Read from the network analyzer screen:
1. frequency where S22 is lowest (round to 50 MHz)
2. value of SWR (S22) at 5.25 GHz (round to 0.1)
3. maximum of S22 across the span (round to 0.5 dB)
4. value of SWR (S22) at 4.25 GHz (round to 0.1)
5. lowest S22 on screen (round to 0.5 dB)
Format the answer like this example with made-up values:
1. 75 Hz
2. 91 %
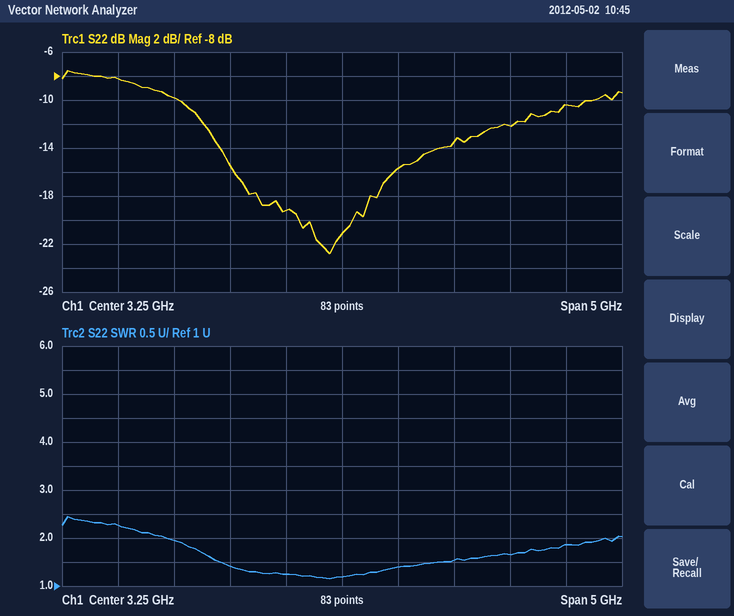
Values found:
1. 3.15 GHz
2. 1.9
3. -7.5 dB
4. 1.5
5. -23.0 dB
